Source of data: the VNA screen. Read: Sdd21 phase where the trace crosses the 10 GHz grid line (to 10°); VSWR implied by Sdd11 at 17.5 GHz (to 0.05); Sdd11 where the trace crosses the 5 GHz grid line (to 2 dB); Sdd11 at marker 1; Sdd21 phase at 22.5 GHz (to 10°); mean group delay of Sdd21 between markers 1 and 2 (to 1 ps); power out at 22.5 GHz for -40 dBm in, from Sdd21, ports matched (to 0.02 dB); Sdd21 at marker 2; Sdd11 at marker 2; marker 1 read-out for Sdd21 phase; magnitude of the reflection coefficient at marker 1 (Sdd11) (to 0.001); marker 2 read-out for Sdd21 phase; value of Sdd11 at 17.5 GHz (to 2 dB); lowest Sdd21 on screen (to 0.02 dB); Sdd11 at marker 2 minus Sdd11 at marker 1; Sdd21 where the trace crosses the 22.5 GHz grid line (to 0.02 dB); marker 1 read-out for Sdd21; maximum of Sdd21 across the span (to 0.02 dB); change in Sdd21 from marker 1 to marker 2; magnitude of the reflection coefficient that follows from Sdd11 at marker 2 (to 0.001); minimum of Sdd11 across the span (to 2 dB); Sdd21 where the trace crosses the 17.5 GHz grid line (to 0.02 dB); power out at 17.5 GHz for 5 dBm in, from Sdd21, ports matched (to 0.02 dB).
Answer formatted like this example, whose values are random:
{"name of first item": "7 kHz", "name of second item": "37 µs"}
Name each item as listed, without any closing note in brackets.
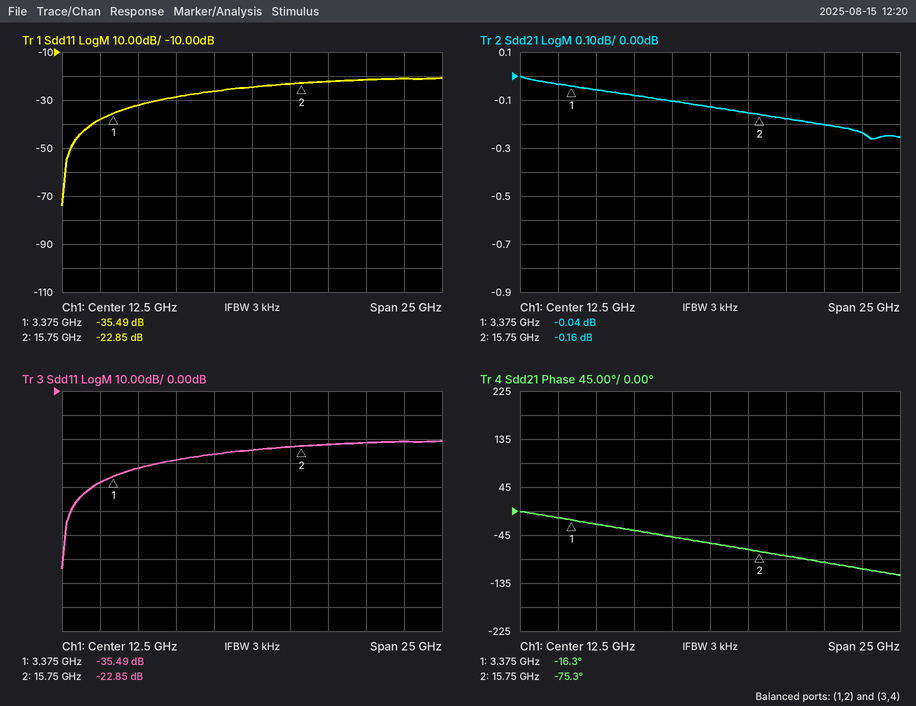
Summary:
{"Sdd21 phase where the trace crosses the 10 GHz grid line": "-50°", "VSWR implied by Sdd11 at 17.5 GHz": "1.15", "Sdd11 where the trace crosses the 5 GHz grid line": "-32 dB", "Sdd11 at marker 1": "-35.49 dB", "Sdd21 phase at 22.5 GHz": "-110°", "mean group delay of Sdd21 between markers 1 and 2": "13 ps", "power out at 22.5 GHz for -40 dBm in, from Sdd21, ports matched": "-40.24 dBm", "Sdd21 at marker 2": "-0.16 dB", "Sdd11 at marker 2": "-22.85 dB", "marker 1 read-out for Sdd21 phase": "-16.3°", "magnitude of the reflection coefficient at marker 1 (Sdd11)": "0.017", "marker 2 read-out for Sdd21 phase": "-75.3°", "value of Sdd11 at 17.5 GHz": "-22 dB", "lowest Sdd21 on screen": "-0.26 dB", "Sdd11 at marker 2 minus Sdd11 at marker 1": "12.64 dB", "Sdd21 where the trace crosses the 22.5 GHz grid line": "-0.24 dB", "marker 1 read-out for Sdd21": "-0.04 dB", "maximum of Sdd21 across the span": "0.00 dB", "change in Sdd21 from marker 1 to marker 2": "-0.12 dB", "magnitude of the reflection coefficient that follows from Sdd11 at marker 2": "0.072", "minimum of Sdd11 across the span": "-74 dB", "Sdd21 where the trace crosses the 17.5 GHz grid line": "-0.18 dB", "power out at 17.5 GHz for 5 dBm in, from Sdd21, ports matched": "4.82 dBm"}
